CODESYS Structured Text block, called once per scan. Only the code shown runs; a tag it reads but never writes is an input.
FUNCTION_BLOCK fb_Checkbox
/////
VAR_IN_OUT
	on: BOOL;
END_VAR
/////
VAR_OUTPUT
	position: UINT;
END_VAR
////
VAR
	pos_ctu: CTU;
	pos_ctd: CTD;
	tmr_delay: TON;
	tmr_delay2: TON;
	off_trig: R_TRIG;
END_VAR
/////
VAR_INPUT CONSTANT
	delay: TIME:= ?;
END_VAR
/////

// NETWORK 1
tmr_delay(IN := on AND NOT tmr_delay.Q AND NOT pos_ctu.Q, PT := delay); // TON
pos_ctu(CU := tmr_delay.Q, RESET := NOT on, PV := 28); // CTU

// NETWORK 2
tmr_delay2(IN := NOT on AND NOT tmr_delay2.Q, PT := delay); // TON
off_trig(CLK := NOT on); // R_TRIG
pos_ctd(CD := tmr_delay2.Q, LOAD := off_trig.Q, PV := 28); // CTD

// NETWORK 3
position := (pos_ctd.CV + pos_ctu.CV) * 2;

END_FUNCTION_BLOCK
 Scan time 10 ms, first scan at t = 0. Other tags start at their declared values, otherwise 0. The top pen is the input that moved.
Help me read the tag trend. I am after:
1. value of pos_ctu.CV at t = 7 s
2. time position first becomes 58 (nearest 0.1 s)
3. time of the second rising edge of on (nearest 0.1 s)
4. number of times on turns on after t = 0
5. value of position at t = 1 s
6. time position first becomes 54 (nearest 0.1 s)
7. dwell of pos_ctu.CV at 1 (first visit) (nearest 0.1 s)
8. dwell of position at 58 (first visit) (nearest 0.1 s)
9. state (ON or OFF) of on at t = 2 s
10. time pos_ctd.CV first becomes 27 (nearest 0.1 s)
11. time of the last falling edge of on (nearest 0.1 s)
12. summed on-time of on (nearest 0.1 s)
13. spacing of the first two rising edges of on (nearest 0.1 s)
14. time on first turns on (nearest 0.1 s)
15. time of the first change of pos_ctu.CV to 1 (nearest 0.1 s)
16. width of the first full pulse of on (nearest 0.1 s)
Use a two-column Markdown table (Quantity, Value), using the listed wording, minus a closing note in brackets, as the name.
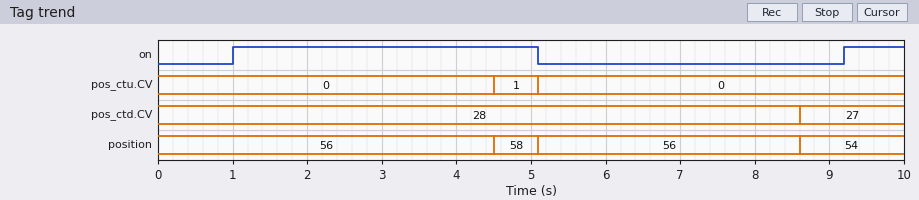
| Quantity | Value |
|---|---|
| value of pos_ctu.CV at t = 7 s | 0 |
| time position first becomes 58 | 4.5 s |
| time of the second rising edge of on | 9.2 s |
| number of times on turns on after t = 0 | 2 |
| value of position at t = 1 s | 56 |
| time position first becomes 54 | 8.6 s |
| dwell of pos_ctu.CV at 1 (first visit) | 0.6 s |
| dwell of position at 58 (first visit) | 0.6 s |
| state (ON or OFF) of on at t = 2 s | ON |
| time pos_ctd.CV first becomes 27 | 8.6 s |
| time of the last falling edge of on | 5.1 s |
| summed on-time of on | 4.9 s |
| spacing of the first two rising edges of on | 8.2 s |
| time on first turns on | 1.0 s |
| time of the first change of pos_ctu.CV to 1 | 4.5 s |
| width of the first full pulse of on | 4.1 s |
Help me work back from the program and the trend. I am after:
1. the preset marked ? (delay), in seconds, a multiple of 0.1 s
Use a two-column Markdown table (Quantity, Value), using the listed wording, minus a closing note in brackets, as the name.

| Quantity | Value |
|---|---|
| the preset marked ? (delay), in seconds, a multiple of 0.1 s | 3.5 s |
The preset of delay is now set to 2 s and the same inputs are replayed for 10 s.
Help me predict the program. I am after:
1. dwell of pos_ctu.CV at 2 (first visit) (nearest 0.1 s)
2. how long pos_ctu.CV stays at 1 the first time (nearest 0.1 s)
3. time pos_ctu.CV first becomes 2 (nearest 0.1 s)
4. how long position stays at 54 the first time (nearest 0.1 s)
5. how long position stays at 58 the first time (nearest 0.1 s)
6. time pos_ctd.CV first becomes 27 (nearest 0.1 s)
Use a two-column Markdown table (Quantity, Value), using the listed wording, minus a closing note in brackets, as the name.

| Quantity | Value |
|---|---|
| dwell of pos_ctu.CV at 2 (first visit) | 0.1 s |
| how long pos_ctu.CV stays at 1 the first time | 2.0 s |
| time pos_ctu.CV first becomes 2 | 5.0 s |
| how long position stays at 54 the first time | 2.0 s |
| how long position stays at 58 the first time | 2.0 s |
| time pos_ctd.CV first becomes 27 | 7.1 s |
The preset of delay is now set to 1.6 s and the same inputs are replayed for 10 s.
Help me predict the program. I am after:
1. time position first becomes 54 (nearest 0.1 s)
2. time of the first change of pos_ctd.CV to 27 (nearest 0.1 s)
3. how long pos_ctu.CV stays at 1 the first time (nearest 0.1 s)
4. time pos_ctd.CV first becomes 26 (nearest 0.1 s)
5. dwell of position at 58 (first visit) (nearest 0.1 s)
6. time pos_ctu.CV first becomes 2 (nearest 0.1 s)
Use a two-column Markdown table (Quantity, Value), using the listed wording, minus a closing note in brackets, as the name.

| Quantity | Value |
|---|---|
| time position first becomes 54 | 6.7 s |
| time of the first change of pos_ctd.CV to 27 | 6.7 s |
| how long pos_ctu.CV stays at 1 the first time | 1.6 s |
| time pos_ctd.CV first becomes 26 | 8.3 s |
| dwell of position at 58 (first visit) | 1.6 s |
| time pos_ctu.CV first becomes 2 | 4.2 s |
